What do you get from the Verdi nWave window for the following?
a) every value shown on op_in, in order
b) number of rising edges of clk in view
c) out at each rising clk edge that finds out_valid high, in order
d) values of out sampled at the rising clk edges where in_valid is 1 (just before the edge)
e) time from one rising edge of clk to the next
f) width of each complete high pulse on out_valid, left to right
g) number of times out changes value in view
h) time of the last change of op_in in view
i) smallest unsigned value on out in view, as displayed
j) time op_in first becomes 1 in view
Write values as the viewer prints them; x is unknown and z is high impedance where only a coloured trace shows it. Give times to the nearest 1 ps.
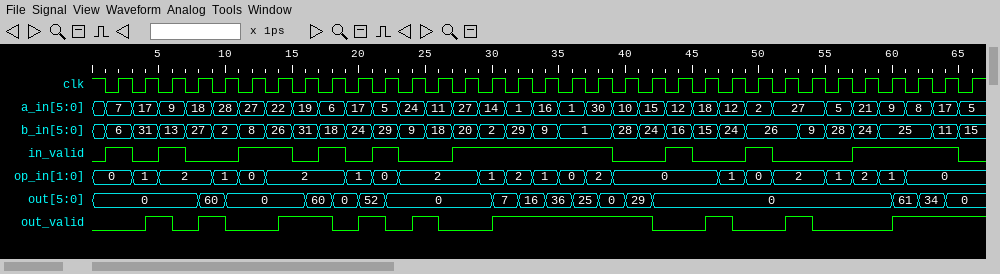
0, 1, 2, 1, 0, 2, 1, 0, 2, 1, 2, 1, 0, 2, 0, 1, 0, 2, 1, 2, 1, 0
33
0, 60, 0, 60, 52, 0, 7, 16, 36, 25, 0, 29, 0, 0, 61, 34, 0
0, 0, 0, 0, 60, 52, 0, 0, 7, 16, 36, 25, 0, 0, 0, 0, 61, 34
2 ps
2 ps, 2 ps, 4 ps, 2 ps, 2 ps, 12 ps, 2 ps, 2 ps
16
61 ps
0
3 ps
